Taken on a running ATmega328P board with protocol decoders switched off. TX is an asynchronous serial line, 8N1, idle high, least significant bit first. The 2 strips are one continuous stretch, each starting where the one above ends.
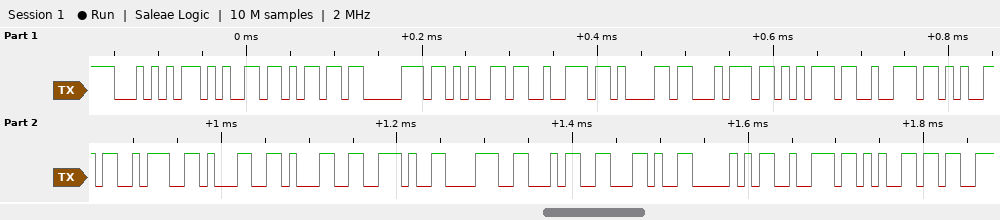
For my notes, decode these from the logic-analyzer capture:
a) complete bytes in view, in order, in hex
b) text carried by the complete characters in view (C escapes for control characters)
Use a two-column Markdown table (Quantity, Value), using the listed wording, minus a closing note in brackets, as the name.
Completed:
| Quantity | Value |
|---|---|
| complete bytes in view, in order, in hex | 54 65 6D 70 65 72 61 74 75 72 65 3A 31 31 2E 38 34 2C 50 72 65 |
| text carried by the complete characters in view | "Temperature:11.84,Pre" |
